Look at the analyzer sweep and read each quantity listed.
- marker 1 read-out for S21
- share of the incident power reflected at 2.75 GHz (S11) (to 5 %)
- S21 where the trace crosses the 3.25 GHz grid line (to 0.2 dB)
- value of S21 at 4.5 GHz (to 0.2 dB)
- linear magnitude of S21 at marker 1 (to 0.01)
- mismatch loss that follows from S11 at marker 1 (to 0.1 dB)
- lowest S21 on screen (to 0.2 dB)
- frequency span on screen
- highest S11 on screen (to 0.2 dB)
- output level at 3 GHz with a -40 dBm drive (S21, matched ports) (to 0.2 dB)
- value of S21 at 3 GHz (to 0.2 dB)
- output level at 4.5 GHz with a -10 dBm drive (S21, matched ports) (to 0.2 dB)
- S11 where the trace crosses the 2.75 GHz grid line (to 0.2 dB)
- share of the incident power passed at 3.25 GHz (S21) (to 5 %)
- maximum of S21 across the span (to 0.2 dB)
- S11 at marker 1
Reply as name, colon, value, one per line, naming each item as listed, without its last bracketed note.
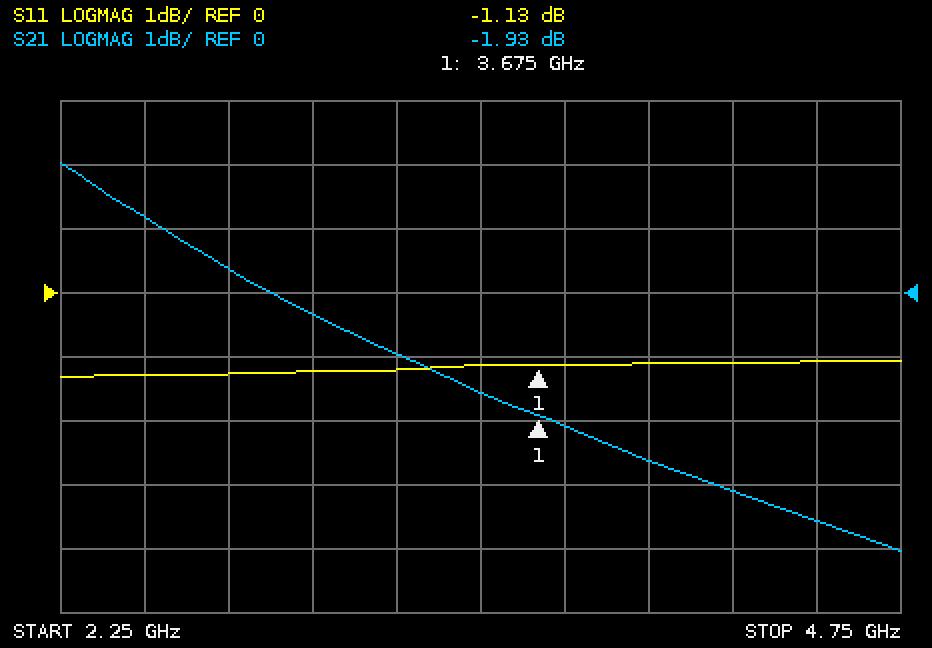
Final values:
marker 1 read-out for S21: -1.93 dB
share of the incident power reflected at 2.75 GHz (S11): 75 %
S21 where the trace crosses the 3.25 GHz grid line: -1.0 dB
value of S21 at 4.5 GHz: -3.6 dB
linear magnitude of S21 at marker 1: 0.80
mismatch loss that follows from S11 at marker 1: 6.4 dB
lowest S21 on screen: -4.0 dB
frequency span on screen: 2.5 GHz
highest S11 on screen: -1.0 dB
output level at 3 GHz with a -40 dBm drive (S21, matched ports): -40.4 dBm
value of S21 at 3 GHz: -0.4 dB
output level at 4.5 GHz with a -10 dBm drive (S21, matched ports): -13.6 dBm
S11 where the trace crosses the 2.75 GHz grid line: -1.2 dB
share of the incident power passed at 3.25 GHz (S21): 80 %
maximum of S21 across the span: 2.0 dB
S11 at marker 1: -1.13 dB
